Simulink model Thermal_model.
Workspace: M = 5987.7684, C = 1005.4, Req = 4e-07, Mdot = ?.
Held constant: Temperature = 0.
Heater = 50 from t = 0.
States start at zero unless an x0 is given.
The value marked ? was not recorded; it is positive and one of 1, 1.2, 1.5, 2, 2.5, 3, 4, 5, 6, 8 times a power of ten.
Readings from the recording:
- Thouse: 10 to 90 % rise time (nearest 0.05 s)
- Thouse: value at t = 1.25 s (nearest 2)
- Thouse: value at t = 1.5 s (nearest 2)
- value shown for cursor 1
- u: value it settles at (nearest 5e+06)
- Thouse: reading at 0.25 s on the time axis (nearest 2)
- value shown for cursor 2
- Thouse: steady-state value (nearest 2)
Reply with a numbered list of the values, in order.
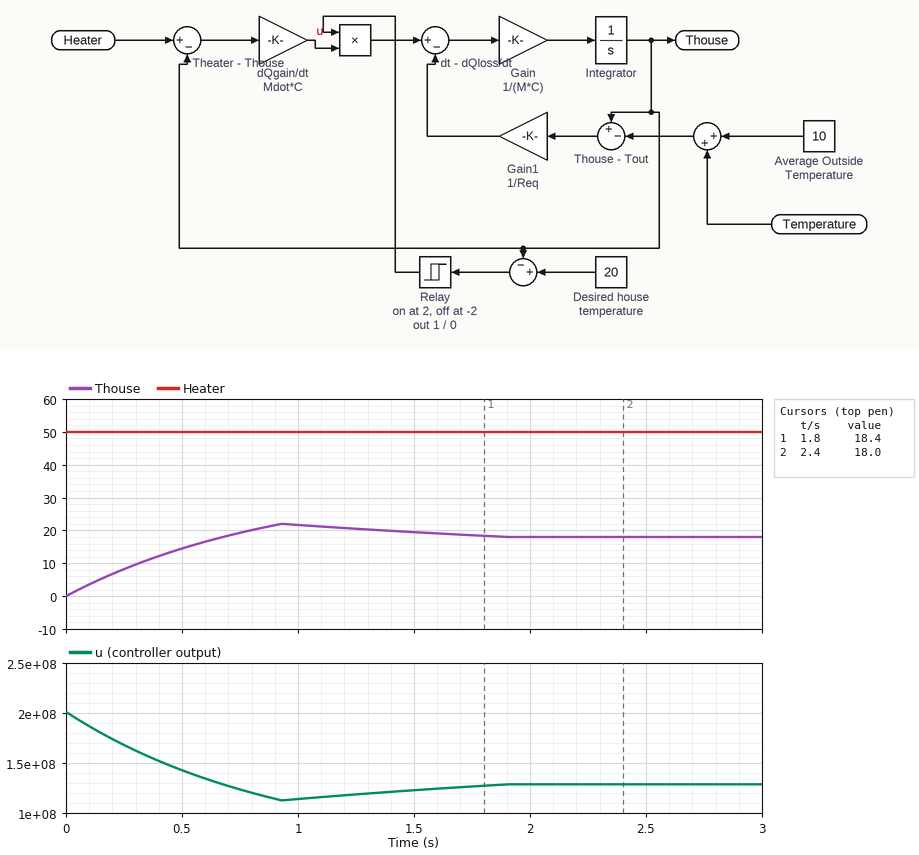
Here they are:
1. 0.55 s
2. 20
3. 20
4. 18.4
5. 130000000
6. 8
7. 18.0
8. 18
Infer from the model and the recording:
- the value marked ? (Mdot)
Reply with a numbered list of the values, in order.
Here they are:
1. 4000
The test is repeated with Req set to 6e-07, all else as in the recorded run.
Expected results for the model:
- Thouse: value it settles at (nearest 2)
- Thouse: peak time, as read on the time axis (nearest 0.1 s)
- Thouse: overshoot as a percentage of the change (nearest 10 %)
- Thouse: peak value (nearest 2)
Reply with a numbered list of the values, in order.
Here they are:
1. 18
2. 0.9 s
3. 20 %
4. 22
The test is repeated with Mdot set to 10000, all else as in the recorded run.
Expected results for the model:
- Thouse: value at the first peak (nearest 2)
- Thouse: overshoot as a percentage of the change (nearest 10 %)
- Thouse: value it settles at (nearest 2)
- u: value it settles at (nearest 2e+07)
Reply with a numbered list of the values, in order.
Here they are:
1. 22
2. 20 %
3. 18
4. 320000000
